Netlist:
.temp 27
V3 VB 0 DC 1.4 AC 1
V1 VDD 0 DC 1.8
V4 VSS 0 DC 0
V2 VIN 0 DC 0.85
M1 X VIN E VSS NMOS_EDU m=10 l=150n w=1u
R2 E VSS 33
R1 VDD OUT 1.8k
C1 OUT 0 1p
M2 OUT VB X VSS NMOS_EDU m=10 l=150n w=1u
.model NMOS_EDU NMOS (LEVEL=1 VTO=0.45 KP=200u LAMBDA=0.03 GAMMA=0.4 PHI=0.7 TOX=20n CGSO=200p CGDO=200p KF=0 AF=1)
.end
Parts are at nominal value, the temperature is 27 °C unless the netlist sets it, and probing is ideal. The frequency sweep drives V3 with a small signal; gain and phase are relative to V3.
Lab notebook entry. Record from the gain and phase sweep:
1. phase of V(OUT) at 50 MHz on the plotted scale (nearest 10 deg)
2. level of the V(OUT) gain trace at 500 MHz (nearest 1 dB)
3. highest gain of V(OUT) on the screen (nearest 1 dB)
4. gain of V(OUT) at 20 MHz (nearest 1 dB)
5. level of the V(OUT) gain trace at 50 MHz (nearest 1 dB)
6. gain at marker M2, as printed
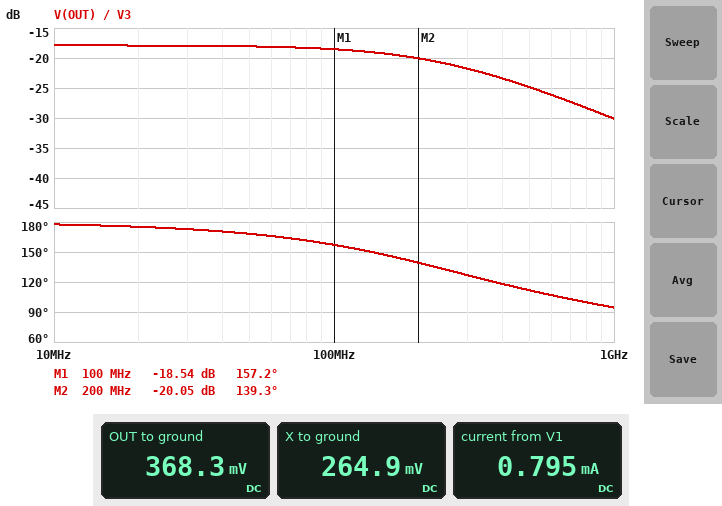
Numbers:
170 deg
-25 dB
-18 dB
-18 dB
-18 dB
-20.05 dB
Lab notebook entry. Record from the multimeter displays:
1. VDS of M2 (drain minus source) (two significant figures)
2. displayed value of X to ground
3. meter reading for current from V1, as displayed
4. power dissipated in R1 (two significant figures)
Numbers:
100 mV
264.9 mV
0.795 mA
1.1 mW
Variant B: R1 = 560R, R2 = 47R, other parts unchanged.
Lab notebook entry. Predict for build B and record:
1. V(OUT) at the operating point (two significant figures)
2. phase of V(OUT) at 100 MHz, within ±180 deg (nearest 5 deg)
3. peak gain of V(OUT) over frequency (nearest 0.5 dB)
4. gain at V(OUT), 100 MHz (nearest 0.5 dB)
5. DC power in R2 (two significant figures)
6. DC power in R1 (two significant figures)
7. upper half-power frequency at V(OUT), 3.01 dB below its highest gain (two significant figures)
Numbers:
1.3 V
160 deg
-41.0 dB
-41.5 dB
33 µW
390 µW
290 MHz
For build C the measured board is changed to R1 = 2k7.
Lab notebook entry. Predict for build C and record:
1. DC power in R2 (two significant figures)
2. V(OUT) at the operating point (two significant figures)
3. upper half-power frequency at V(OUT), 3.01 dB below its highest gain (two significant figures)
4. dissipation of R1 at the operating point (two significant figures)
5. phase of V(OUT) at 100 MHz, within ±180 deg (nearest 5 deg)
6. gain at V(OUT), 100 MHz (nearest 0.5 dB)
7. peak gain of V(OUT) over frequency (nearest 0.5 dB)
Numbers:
11 µW
220 mV
360 MHz
920 µW
165 deg
-23.0 dB
-22.5 dB
